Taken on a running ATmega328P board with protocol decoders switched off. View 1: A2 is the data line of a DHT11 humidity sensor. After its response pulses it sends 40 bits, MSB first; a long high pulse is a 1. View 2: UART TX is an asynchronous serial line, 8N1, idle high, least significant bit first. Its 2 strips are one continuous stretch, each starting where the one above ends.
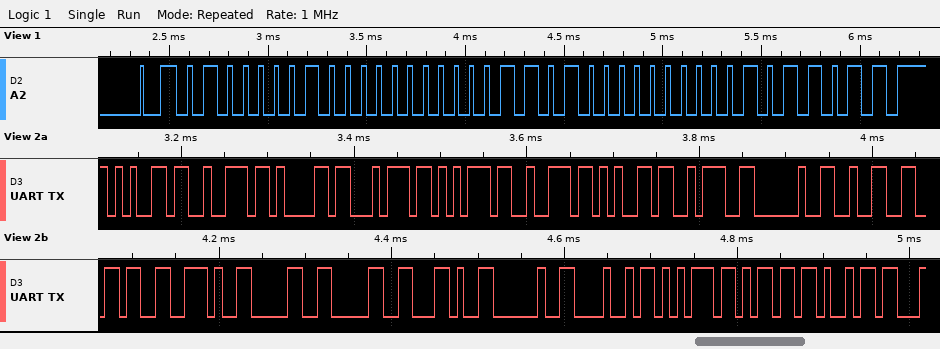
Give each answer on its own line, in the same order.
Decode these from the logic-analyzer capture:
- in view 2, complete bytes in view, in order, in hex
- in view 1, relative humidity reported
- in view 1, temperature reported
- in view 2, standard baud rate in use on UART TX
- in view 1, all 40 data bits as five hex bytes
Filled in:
65 72 61 74 75 72 65 3A 20 32 36 2E 30 30 2C 20 48 75 6D 69
65 %
26.0 °C
115200 baud
41 00 1A 00 5B
